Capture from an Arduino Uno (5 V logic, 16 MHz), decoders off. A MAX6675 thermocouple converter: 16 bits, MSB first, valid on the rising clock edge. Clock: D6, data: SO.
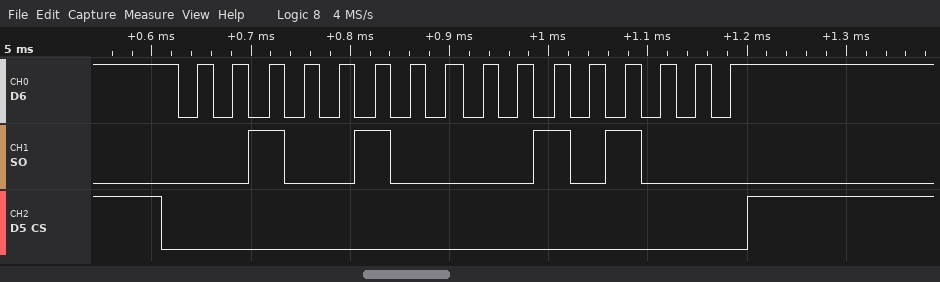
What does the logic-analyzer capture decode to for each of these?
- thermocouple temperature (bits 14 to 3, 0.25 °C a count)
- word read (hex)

289.25 °C
0x2428
